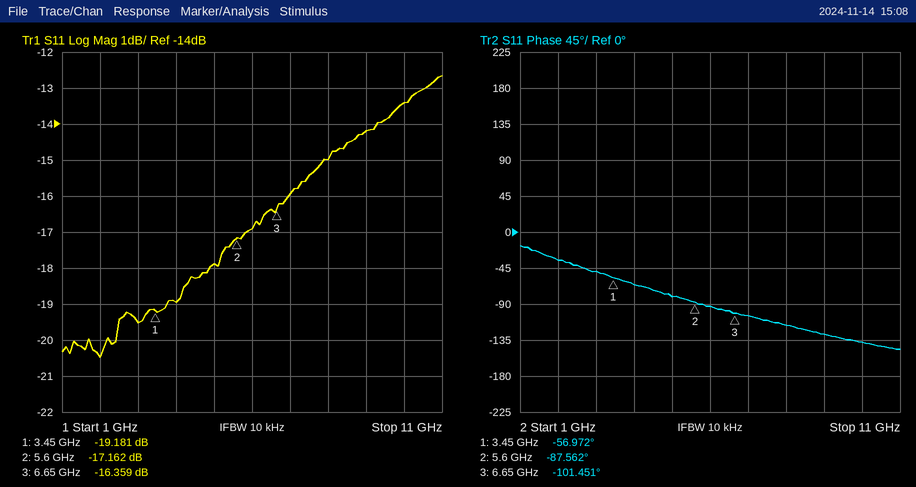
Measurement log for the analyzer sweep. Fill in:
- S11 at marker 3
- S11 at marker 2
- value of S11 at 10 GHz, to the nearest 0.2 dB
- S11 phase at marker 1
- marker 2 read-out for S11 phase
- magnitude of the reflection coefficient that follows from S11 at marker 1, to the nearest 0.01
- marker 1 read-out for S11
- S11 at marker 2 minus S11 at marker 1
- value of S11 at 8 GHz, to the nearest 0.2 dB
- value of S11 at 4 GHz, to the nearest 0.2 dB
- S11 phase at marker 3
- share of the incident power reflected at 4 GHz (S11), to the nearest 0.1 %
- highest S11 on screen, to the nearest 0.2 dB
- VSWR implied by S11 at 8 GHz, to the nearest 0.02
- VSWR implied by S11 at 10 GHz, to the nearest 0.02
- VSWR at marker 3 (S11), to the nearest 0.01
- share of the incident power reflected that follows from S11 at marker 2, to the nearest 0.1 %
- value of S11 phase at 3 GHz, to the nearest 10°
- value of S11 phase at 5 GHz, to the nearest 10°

-16.359 dB
-17.162 dB
-13.4 dB
-56.972°
-87.562°
0.11
-19.181 dB
2.019 dB
-15.0 dB
-19.0 dB
-101.451°
1.3 %
-12.6 dB
1.44
1.54
1.36
1.9 %
-50°
-80°
